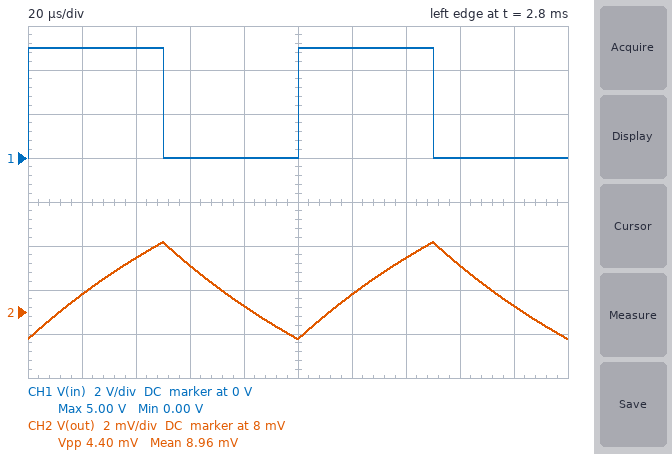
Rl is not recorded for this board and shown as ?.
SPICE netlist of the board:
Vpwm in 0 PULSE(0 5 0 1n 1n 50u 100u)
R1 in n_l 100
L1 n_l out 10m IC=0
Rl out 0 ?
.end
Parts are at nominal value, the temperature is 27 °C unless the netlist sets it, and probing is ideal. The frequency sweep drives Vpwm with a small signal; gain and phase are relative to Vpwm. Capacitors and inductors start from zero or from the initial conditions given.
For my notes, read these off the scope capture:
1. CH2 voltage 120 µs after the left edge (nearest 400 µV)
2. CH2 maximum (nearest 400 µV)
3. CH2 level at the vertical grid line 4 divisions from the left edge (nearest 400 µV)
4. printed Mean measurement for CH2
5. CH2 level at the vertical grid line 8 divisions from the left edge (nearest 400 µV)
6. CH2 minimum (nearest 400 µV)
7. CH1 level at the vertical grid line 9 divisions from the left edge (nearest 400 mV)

8.8 mV
11.2 mV
8.4 mV
8.96 mV
10.0 mV
6.8 mV
0 V
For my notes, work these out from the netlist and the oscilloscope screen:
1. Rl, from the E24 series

0.36 Ω
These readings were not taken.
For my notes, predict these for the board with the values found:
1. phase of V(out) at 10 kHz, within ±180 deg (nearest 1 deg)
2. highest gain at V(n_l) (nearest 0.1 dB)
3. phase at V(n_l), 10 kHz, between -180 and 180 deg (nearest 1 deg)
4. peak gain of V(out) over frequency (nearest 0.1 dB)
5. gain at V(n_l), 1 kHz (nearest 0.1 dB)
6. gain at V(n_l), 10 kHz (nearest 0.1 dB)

-81 deg
0 dB
9 deg
-48.9 dB
-5.5 dB
-0.1 dB
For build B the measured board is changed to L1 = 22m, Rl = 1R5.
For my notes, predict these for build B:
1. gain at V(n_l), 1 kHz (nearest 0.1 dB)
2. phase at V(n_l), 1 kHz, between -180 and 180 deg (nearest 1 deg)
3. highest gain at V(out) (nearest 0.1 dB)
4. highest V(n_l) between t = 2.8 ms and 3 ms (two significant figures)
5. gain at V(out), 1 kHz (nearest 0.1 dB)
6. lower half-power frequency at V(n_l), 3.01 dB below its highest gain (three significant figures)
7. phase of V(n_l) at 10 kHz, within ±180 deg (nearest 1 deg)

-1.9 dB
36 deg
-36.6 dB
2.8 V
-41.2 dB
734 Hz
4 deg
